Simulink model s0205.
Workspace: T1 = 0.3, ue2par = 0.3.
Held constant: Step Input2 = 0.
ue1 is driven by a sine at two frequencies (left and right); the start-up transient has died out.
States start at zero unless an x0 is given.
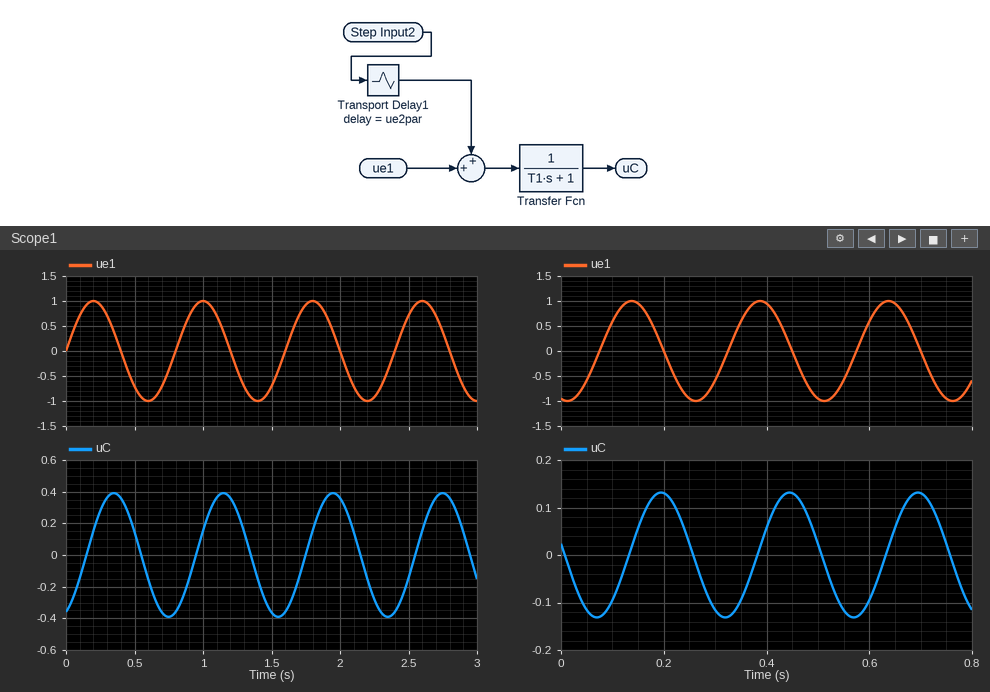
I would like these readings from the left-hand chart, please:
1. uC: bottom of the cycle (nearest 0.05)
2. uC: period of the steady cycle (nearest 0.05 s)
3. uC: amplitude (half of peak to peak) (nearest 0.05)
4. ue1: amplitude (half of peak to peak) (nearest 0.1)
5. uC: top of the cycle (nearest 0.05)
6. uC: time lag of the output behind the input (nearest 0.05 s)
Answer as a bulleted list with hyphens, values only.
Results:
- -0.40
- 0.80 s
- 0.40
- 1.0
- 0.40
- 0.15 s
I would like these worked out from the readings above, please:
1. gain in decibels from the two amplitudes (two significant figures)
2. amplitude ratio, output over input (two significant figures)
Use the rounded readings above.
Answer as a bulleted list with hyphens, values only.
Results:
- -8.0 dB
- 0.40
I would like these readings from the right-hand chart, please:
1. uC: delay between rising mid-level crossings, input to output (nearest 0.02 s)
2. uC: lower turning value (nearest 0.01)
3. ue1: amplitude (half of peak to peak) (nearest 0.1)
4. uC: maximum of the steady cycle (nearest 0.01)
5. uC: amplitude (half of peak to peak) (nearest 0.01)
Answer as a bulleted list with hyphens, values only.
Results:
- 0.06 s
- -0.13
- 1.0
- 0.13
- 0.13
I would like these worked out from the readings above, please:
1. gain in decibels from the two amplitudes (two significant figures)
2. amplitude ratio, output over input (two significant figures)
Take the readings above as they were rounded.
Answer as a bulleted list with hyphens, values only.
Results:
- -18 dB
- 0.13
